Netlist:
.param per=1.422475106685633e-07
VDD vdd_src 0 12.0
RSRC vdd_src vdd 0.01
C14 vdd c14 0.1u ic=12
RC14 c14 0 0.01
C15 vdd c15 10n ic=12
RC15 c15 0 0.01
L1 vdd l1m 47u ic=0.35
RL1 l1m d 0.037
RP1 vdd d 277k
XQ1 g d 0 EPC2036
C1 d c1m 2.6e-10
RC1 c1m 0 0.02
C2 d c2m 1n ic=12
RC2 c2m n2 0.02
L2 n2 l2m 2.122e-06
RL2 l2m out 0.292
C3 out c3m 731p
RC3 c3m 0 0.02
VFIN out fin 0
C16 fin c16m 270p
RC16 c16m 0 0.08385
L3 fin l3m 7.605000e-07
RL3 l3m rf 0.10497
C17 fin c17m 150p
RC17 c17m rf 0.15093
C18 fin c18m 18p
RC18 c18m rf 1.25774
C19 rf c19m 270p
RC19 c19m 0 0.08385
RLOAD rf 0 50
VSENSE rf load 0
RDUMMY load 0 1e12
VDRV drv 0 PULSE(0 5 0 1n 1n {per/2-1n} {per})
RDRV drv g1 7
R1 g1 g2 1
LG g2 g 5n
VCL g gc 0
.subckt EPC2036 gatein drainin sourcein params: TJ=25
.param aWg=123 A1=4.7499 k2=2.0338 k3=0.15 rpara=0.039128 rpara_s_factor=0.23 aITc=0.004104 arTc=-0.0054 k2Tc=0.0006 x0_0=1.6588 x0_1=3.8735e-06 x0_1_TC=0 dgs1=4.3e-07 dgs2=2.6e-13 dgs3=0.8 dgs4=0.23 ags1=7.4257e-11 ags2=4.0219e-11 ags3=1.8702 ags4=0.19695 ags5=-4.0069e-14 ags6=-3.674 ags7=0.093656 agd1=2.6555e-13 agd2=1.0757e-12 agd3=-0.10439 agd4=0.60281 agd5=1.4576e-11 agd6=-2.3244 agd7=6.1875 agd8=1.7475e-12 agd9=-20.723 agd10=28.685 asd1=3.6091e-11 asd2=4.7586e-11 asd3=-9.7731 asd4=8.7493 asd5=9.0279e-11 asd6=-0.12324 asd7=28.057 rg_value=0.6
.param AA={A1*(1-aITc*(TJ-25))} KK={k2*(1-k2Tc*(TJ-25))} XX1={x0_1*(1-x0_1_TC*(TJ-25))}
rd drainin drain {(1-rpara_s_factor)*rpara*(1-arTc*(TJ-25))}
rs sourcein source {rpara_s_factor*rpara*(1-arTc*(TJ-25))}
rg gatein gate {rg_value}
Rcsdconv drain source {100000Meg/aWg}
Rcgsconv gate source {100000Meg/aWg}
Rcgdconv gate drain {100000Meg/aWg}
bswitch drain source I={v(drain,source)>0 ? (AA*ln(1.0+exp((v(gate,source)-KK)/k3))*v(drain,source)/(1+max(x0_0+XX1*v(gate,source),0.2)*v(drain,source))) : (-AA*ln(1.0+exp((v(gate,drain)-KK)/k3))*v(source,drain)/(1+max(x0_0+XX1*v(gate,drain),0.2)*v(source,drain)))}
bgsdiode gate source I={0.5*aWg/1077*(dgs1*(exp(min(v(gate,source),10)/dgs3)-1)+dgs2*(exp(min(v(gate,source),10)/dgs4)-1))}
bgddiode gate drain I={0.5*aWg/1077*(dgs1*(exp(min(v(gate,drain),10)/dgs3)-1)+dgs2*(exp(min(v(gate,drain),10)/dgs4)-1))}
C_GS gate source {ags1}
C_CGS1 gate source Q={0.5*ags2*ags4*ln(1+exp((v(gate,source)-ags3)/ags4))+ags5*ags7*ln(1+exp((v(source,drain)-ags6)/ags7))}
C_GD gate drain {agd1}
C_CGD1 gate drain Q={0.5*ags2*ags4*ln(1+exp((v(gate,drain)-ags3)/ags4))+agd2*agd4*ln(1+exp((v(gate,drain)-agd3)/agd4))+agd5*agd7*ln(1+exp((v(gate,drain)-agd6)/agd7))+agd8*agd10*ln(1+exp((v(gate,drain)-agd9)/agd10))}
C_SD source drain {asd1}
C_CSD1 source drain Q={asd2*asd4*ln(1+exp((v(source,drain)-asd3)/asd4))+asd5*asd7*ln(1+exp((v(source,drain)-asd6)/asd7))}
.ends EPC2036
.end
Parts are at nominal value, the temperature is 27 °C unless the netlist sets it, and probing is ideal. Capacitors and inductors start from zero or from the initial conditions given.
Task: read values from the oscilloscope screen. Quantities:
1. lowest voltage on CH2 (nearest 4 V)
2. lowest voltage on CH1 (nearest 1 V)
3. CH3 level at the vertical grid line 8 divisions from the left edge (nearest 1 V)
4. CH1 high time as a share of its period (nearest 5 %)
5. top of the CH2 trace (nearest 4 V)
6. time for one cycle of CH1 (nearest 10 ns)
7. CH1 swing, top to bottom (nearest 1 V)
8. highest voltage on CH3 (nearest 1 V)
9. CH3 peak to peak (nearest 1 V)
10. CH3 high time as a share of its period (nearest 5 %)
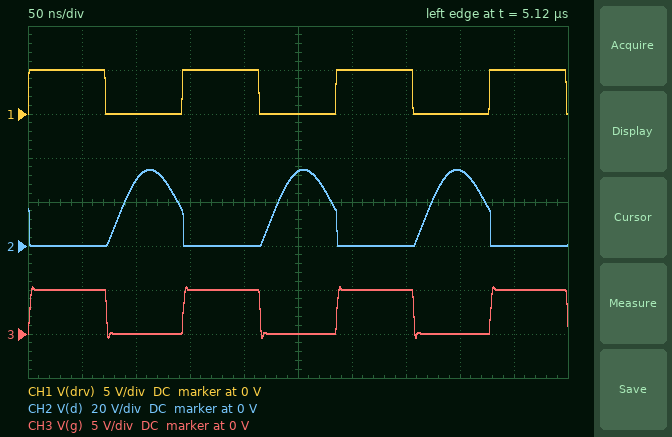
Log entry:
0 V
0 V
0 V
50 %
36 V
140 ns
5 V
5 V
6 V
50 %
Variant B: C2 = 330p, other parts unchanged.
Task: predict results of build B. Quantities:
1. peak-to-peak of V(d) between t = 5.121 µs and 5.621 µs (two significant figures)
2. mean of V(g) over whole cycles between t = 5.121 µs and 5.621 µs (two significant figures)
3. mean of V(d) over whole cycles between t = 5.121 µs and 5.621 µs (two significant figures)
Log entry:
30 V
2.5 V
10 V
